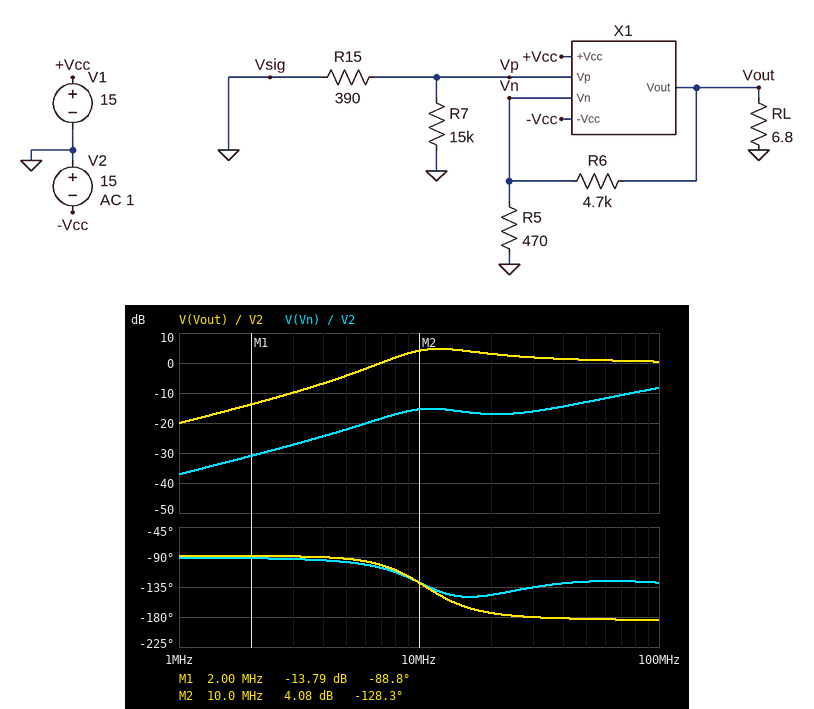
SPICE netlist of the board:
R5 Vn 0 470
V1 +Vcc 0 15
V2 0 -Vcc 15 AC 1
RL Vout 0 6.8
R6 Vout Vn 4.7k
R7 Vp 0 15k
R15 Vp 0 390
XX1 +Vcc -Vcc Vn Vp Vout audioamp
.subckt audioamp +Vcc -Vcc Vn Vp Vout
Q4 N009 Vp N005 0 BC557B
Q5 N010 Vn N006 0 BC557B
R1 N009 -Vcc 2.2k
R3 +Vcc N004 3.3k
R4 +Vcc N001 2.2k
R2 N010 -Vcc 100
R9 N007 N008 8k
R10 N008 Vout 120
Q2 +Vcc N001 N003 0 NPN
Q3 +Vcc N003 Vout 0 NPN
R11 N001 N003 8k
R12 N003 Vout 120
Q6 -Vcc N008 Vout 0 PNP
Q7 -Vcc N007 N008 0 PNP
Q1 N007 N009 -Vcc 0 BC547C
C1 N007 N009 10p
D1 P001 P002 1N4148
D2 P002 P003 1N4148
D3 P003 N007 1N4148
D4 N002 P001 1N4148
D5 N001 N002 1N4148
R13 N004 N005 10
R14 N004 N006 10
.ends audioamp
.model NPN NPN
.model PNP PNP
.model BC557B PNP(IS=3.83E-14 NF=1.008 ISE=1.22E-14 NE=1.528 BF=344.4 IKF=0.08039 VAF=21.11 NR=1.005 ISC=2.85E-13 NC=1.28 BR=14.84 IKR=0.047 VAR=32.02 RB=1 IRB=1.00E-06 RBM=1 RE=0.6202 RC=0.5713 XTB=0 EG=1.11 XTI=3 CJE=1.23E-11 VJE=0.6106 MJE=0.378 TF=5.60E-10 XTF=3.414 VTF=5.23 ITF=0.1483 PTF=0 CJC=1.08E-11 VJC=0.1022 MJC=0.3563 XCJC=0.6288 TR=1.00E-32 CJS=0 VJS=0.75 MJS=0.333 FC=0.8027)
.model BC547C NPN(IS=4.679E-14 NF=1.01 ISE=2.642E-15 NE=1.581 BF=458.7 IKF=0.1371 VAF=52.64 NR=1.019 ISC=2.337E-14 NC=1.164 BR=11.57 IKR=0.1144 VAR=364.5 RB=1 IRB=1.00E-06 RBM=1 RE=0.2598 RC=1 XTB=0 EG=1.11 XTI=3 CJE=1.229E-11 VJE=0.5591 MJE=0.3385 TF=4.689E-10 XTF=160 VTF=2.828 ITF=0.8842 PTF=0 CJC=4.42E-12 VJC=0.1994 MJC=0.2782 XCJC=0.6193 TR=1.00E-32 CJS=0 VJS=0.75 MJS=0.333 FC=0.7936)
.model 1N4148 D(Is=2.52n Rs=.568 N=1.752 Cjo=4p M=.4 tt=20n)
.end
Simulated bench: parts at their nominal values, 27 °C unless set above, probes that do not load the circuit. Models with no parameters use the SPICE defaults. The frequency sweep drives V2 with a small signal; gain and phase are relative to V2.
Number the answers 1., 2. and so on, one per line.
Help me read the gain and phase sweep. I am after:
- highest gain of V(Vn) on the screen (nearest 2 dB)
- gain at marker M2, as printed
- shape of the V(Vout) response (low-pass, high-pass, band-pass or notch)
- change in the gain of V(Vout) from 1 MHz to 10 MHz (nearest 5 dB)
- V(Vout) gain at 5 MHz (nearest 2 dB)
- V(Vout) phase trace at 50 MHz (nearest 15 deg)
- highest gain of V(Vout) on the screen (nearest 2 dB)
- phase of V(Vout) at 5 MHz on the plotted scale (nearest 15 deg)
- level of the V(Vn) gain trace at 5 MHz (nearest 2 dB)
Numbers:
1. -8 dB
2. 4.08 dB
3. high-pass
4. 25 dB
5. -4 dB
6. -180 deg
7. 4 dB
8. -90 deg
9. -22 dB
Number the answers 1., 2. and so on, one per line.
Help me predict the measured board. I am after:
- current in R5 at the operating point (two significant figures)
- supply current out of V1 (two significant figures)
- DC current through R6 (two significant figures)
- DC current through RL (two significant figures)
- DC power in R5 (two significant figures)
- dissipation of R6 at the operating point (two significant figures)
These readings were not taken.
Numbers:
1. 230 µA
2. 20 mA
3. 230 µA
4. 180 mA
5. 24 µW
6. 260 µW
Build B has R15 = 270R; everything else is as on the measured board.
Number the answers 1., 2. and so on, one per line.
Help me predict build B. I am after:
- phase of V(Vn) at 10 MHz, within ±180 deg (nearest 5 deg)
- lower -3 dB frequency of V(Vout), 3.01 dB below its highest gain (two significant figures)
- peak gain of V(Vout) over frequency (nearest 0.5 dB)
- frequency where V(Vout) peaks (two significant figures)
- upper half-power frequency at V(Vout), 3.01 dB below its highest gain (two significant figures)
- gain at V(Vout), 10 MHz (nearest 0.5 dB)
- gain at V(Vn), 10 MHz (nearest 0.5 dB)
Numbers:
1. -120 deg
2. 8.9 MHz
3. 4.0 dB
4. 14 MHz
5. 74 MHz
6. 2.0 dB
7. -16.5 dB
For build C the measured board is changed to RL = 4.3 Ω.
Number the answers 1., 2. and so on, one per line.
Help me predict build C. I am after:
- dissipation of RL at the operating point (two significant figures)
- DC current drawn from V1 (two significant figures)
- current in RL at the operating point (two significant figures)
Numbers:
1. 340 mW
2. 19 mA
3. 280 mA
